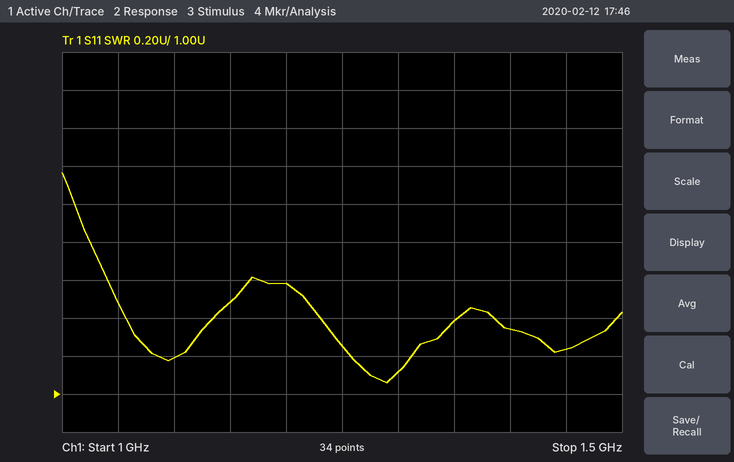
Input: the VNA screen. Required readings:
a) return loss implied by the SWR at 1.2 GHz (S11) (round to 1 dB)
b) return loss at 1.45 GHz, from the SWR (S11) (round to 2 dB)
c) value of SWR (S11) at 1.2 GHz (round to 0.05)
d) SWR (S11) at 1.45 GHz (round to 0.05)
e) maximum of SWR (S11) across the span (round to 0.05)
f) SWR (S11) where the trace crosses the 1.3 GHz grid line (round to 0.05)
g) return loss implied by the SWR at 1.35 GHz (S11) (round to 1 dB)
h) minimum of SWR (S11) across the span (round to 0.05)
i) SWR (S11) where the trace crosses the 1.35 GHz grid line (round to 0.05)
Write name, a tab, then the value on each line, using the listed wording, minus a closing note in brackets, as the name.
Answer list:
return loss implied by the SWR at 1.2 GHz (S11)	13 dB
return loss at 1.45 GHz, from the SWR (S11)	20 dB
value of SWR (S11) at 1.2 GHz	1.60
SWR (S11) at 1.45 GHz	1.25
maximum of SWR (S11) across the span	2.15
SWR (S11) where the trace crosses the 1.3 GHz grid line	1.10
return loss implied by the SWR at 1.35 GHz (S11)	16 dB
minimum of SWR (S11) across the span	1.05
SWR (S11) where the trace crosses the 1.35 GHz grid line	1.40
